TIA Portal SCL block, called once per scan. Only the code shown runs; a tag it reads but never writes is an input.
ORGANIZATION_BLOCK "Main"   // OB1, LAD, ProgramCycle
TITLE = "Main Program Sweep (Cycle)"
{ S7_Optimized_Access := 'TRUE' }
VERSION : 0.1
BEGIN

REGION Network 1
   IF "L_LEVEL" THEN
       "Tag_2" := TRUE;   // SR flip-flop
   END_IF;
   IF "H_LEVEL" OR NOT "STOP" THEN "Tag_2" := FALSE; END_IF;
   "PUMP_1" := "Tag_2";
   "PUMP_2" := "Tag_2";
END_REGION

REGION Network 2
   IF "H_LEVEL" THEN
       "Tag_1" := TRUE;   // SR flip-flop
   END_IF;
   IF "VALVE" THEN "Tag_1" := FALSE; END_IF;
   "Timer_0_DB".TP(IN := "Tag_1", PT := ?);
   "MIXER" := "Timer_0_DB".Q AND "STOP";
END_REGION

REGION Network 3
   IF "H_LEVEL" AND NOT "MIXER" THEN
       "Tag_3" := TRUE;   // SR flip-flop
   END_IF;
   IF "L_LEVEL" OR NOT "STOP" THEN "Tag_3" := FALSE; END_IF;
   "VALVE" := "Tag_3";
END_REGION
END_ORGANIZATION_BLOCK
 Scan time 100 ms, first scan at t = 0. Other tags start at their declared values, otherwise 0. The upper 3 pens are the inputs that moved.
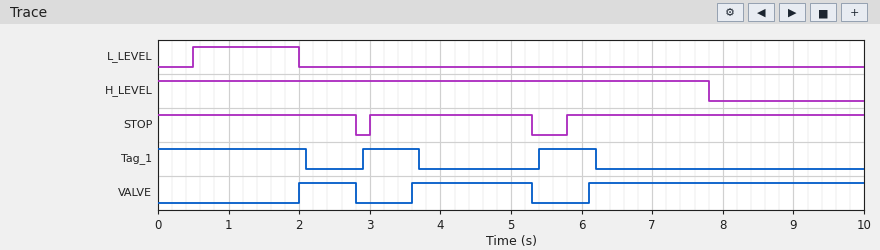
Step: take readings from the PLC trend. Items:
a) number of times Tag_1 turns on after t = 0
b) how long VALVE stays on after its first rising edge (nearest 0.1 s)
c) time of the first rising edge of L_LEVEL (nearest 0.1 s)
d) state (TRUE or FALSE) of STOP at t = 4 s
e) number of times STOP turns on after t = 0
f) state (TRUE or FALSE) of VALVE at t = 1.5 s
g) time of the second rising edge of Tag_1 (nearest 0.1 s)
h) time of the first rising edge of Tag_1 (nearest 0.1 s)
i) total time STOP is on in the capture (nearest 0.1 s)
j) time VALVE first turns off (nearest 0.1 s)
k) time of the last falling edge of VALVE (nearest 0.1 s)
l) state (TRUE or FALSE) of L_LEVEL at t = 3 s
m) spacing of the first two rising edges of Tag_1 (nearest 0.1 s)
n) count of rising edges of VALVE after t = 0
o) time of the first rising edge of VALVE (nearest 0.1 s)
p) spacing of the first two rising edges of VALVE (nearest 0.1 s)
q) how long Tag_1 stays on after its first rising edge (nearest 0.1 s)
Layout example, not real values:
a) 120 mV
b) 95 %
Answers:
a) 2
b) 0.8 s
c) 0.5 s
d) TRUE
e) 2
f) FALSE
g) 5.4 s
h) 2.9 s
i) 9.3 s
j) 2.8 s
k) 5.3 s
l) FALSE
m) 2.5 s
n) 3
o) 2.0 s
p) 1.6 s
q) 0.8 s
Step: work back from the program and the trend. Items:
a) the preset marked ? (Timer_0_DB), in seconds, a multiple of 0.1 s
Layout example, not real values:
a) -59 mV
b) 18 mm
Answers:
a) 0.7 s
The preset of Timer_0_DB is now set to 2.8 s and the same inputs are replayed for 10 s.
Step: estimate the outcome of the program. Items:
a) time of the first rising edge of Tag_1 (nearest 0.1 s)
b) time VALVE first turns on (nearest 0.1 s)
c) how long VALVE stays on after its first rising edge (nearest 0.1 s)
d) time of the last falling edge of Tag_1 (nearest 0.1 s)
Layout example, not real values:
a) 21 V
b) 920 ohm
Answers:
a) 5.4 s
b) 3.0 s
c) 2.3 s
d) 3.1 s
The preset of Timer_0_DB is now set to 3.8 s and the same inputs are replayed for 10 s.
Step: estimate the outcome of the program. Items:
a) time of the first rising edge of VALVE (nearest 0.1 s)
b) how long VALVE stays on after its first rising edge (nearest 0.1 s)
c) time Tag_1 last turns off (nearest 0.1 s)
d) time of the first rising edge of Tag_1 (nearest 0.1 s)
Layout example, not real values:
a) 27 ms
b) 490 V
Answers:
a) 3.8 s
b) 1.5 s
c) 3.9 s
d) 5.4 s
